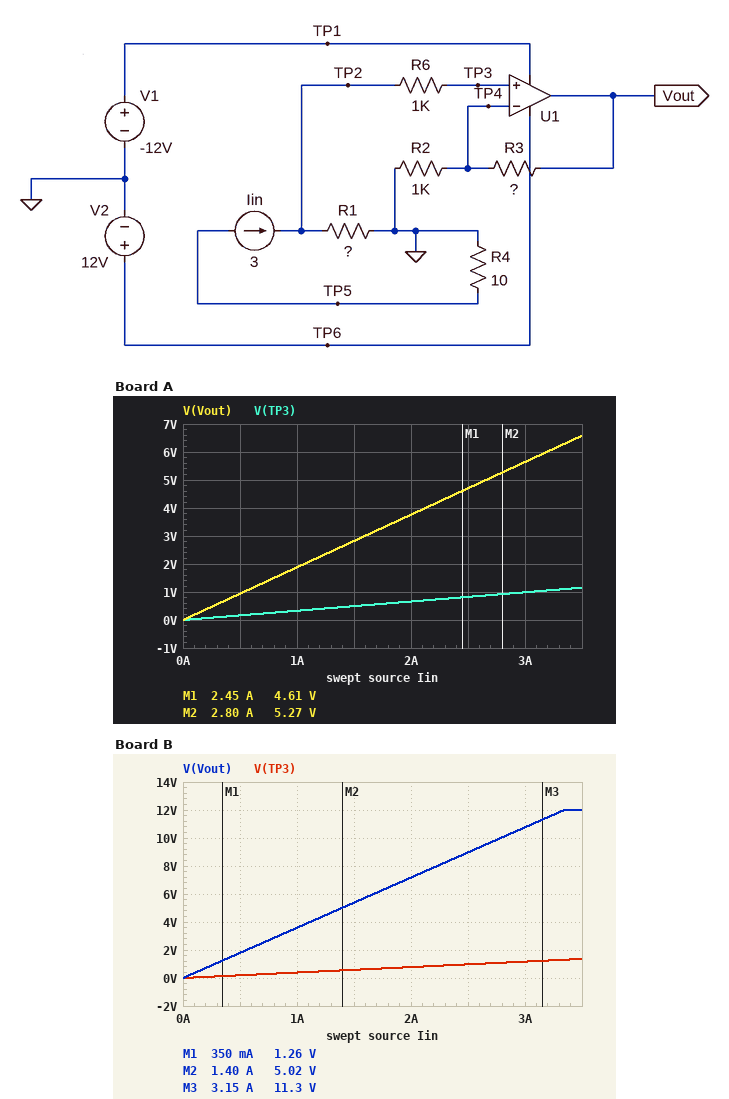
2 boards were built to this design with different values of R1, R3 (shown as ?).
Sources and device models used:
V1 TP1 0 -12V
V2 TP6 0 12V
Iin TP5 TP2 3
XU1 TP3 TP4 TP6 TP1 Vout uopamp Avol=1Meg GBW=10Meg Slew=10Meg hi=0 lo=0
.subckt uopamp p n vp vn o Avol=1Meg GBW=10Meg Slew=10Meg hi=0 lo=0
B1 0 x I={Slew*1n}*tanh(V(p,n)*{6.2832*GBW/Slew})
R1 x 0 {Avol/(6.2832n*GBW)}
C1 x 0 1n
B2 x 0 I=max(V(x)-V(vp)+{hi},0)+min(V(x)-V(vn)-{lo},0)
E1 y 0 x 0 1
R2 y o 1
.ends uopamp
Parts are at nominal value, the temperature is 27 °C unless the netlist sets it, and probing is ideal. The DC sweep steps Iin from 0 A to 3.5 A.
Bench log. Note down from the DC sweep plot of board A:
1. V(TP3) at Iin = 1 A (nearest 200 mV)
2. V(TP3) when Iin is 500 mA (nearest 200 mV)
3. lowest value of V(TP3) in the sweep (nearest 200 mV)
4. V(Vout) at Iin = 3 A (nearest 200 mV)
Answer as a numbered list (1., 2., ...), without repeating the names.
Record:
1. 400 mV
2. 200 mV
3. 0 V
4. 5.6 V
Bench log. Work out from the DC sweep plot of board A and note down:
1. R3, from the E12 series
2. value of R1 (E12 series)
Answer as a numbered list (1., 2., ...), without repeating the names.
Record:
1. 4.7 kΩ
2. 0.33 Ω
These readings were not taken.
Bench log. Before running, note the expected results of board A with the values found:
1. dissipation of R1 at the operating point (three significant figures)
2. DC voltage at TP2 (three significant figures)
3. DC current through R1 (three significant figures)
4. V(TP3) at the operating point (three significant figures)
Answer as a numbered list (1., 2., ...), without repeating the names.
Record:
1. 2.97 W
2. 990 mV
3. 3.00 A
4. 990 mV
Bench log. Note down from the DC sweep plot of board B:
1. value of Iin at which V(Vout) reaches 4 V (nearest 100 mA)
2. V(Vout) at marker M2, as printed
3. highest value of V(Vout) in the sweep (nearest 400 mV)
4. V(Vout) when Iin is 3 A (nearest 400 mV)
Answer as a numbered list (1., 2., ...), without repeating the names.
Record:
1. 1.1 A
2. 5.02 V
3. 12.0 V
4. 10.8 V
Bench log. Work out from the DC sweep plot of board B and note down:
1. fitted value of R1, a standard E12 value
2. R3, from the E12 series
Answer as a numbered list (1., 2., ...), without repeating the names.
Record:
1. 0.39 Ω
2. 8.2 kΩ
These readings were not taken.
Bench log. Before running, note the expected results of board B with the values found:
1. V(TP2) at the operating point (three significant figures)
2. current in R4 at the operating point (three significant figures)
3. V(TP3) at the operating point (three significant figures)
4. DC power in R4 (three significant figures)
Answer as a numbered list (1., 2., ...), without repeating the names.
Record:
1. 1.17 V
2. 3.00 A
3. 1.17 V
4. 90.0 W
